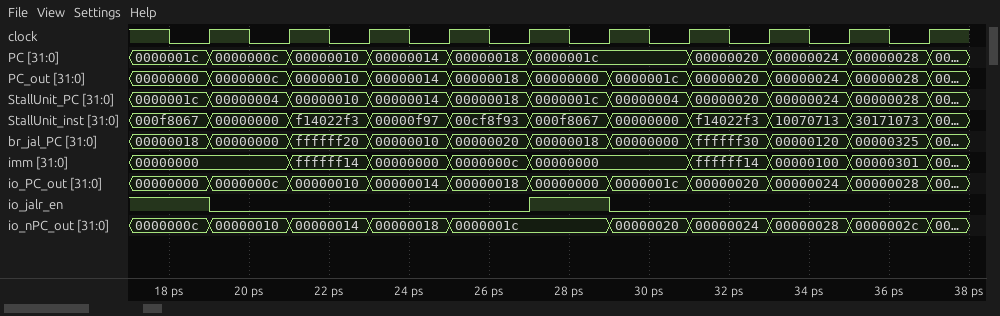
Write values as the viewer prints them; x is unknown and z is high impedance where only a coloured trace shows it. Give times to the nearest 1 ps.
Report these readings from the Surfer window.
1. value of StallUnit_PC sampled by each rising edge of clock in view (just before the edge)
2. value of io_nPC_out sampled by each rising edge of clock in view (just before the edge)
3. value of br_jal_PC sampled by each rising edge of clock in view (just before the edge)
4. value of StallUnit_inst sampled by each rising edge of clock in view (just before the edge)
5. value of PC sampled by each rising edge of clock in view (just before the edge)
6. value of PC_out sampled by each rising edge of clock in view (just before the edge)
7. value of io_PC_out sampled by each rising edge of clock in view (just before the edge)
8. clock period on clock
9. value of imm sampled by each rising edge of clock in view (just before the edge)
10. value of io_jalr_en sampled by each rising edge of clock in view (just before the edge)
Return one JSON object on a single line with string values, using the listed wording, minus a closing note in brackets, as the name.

{"value of StallUnit_PC sampled by each rising edge of clock in view": "0000001c, 00000004, 00000010, 00000014, 00000018, 0000001c, 00000004, 00000020, 00000024, 00000028", "value of io_nPC_out sampled by each rising edge of clock in view": "0000000c, 00000010, 00000014, 00000018, 0000001c, 0000001c, 00000020, 00000024, 00000028, 0000002c", "value of br_jal_PC sampled by each rising edge of clock in view": "00000018, 00000000, ffffff20, 00000010, 00000020, 00000018, 00000000, ffffff30, 00000120, 00000325", "value of StallUnit_inst sampled by each rising edge of clock in view": "000f8067, 00000000, f14022f3, 00000f97, 00cf8f93, 000f8067, 00000000, f14022f3, 10070713, 30171073", "value of PC sampled by each rising edge of clock in view": "0000001c, 0000000c, 00000010, 00000014, 00000018, 0000001c, 0000001c, 00000020, 00000024, 00000028", "value of PC_out sampled by each rising edge of clock in view": "00000000, 0000000c, 00000010, 00000014, 00000018, 00000000, 0000001c, 00000020, 00000024, 00000028", "value of io_PC_out sampled by each rising edge of clock in view": "00000000, 0000000c, 00000010, 00000014, 00000018, 00000000, 0000001c, 00000020, 00000024, 00000028", "clock period on clock": "2 ps", "value of imm sampled by each rising edge of clock in view": "00000000, 00000000, ffffff14, 00000000, 0000000c, 00000000, 00000000, ffffff14, 00000100, 00000301", "value of io_jalr_en sampled by each rising edge of clock in view": "1 0 0 0 0 1 0 0 0 0"}
